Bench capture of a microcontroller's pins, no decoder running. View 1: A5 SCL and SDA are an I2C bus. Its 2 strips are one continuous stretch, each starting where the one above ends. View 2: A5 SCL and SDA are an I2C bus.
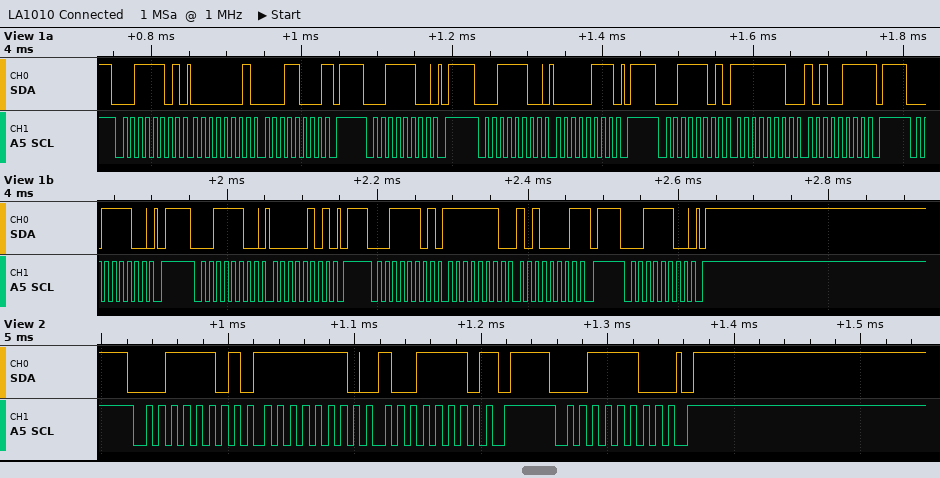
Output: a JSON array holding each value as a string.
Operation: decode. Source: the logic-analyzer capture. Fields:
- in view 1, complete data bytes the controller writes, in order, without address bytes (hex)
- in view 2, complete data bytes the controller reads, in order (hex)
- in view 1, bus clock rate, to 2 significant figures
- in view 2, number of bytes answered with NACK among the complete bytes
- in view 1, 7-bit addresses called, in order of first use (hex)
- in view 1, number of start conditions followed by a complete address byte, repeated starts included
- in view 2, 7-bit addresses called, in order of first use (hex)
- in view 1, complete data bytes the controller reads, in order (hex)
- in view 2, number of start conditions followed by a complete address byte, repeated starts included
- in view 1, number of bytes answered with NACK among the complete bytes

["07 05", "FE 9E", "100 kHz", "1", "0x1E", "8", "0x1E", "01 18 FE A7 FE A1", "2", "3"]
